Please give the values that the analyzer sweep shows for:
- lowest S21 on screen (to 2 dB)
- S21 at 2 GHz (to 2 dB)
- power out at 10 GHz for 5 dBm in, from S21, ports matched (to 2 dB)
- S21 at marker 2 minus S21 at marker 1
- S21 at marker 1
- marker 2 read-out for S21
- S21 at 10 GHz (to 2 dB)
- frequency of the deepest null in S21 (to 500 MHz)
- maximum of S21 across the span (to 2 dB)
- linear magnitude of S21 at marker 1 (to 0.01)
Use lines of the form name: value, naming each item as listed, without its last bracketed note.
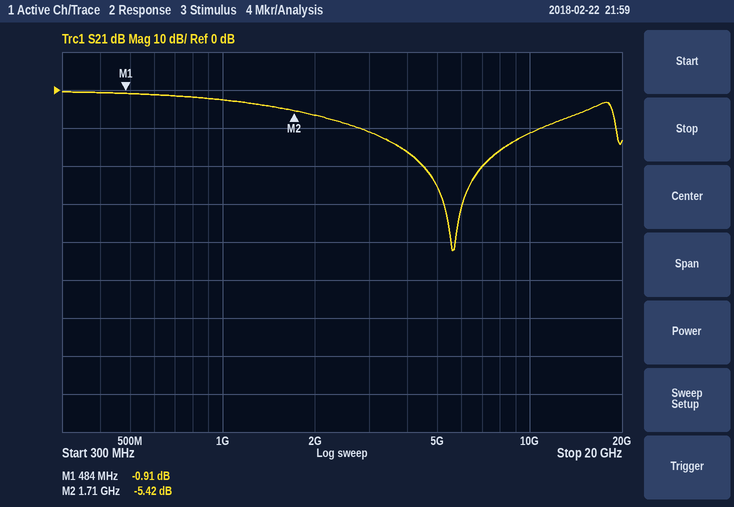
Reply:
lowest S21 on screen: -42 dB
S21 at 2 GHz: -6 dB
power out at 10 GHz for 5 dBm in, from S21, ports matched: -6 dBm
S21 at marker 2 minus S21 at marker 1: -4.51 dB
S21 at marker 1: -0.91 dB
marker 2 read-out for S21: -5.42 dB
S21 at 10 GHz: -12 dB
frequency of the deepest null in S21: 5.5 GHz
maximum of S21 across the span: 0 dB
linear magnitude of S21 at marker 1: 0.90
